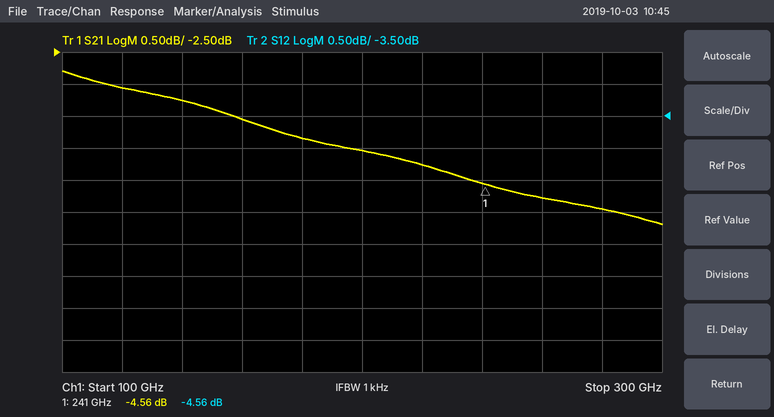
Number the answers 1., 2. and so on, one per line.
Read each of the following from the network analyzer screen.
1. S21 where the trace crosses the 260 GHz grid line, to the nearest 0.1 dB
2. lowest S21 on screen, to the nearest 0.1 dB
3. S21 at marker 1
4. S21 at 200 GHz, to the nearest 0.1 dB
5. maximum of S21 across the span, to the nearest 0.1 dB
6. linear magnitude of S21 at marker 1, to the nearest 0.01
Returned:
1. -4.8 dB
2. -5.2 dB
3. -4.56 dB
4. -4.0 dB
5. -2.8 dB
6. 0.59
